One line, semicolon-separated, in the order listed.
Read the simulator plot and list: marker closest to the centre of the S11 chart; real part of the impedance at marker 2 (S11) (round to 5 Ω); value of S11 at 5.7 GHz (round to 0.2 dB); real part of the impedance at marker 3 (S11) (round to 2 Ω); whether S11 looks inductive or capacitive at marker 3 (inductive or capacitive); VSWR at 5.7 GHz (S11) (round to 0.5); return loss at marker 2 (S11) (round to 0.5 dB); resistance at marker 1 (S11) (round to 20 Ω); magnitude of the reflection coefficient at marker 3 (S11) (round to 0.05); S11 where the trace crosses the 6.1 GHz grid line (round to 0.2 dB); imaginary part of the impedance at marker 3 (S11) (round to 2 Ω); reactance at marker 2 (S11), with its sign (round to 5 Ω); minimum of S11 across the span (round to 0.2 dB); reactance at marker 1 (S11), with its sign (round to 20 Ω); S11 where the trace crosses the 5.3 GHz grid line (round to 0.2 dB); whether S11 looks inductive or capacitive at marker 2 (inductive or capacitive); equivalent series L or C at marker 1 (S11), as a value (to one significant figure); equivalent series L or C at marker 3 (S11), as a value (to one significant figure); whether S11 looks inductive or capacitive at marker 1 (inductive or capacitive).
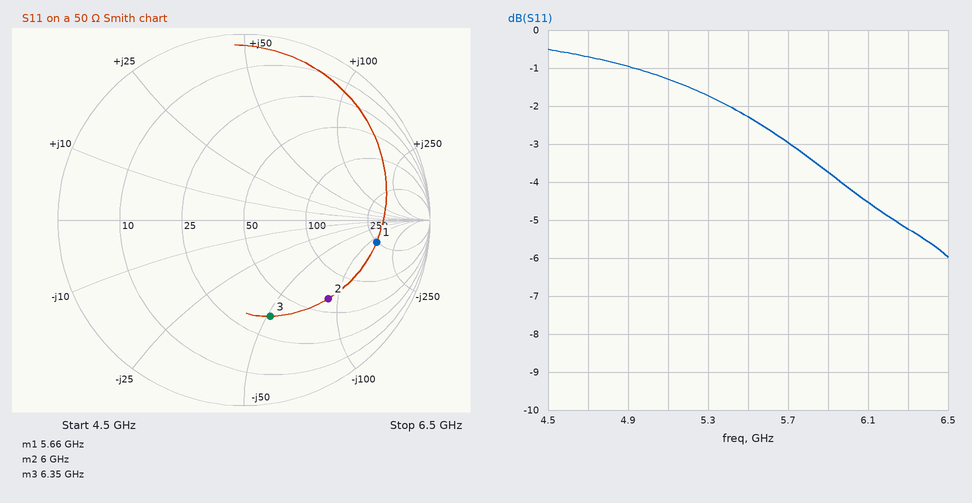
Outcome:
marker 3; 65 Ω; -3.0 dB; 36 Ω; capacitive; 6.0; 4.0 dB; 240 Ω; 0.55; -4.6 dB; -52 Ω; -90 Ω; -6.0 dB; -120 Ω; -1.8 dB; capacitive; 200 fF; 500 fF; capacitive
